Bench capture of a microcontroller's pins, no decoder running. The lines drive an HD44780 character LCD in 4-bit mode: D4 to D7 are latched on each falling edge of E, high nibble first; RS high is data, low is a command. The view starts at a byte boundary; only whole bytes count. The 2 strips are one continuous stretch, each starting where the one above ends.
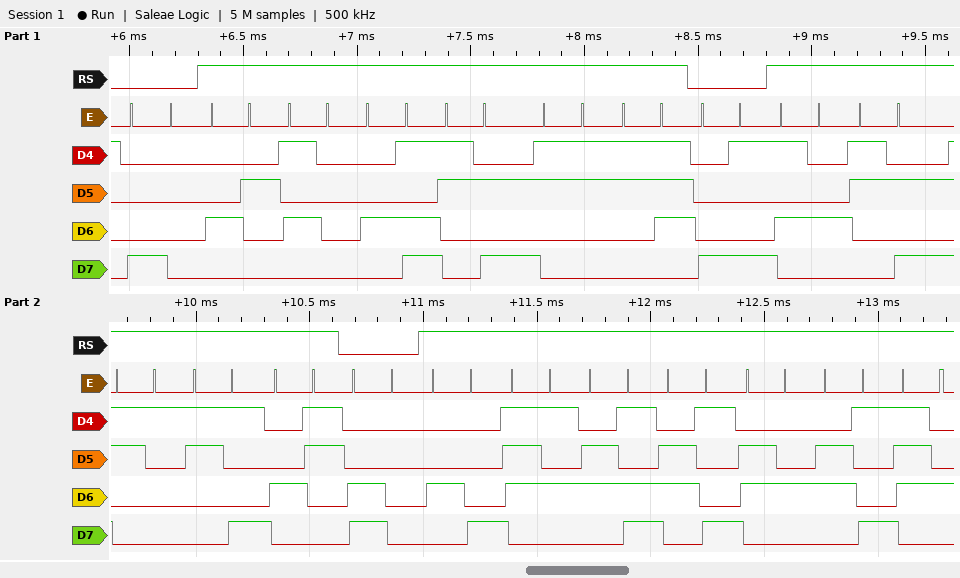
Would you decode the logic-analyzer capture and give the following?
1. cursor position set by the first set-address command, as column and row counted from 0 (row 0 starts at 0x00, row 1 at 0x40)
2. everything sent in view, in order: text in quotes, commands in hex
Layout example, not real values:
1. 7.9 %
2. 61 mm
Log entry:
1. column 0, row 0
2. 0x80 "BPM:37" 0x89 "T:19C" 0xC0 "Humidit"
